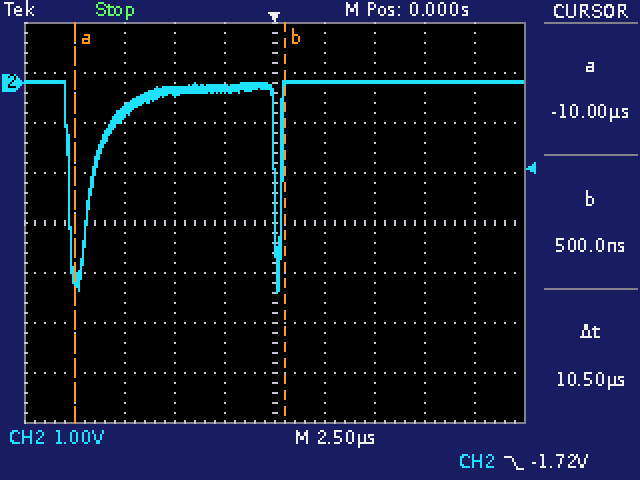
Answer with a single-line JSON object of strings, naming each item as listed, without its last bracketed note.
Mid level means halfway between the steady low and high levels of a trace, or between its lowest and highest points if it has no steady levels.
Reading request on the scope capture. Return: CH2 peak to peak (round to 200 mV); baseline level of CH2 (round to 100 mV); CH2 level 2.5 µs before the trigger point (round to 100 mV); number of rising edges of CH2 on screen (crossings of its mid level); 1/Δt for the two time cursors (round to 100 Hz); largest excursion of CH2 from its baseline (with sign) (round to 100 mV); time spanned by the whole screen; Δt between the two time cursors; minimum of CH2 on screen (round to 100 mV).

{"CH2 peak to peak": "4.2 V", "baseline level of CH2": "0.0 V", "CH2 level 2.5 µs before the trigger point": "-100 mV", "number of rising edges of CH2 on screen": "2", "1/Δt for the two time cursors": "95.2 kHz", "largest excursion of CH2 from its baseline (with sign)": "-4.2 V", "time spanned by the whole screen": "25 µs", "Δt between the two time cursors": "10.5 µs", "minimum of CH2 on screen": "-4.2 V"}
